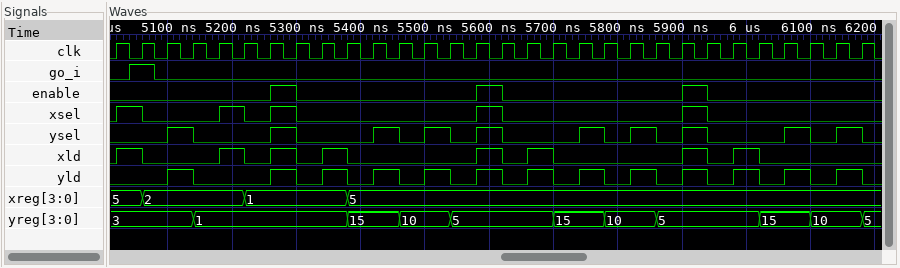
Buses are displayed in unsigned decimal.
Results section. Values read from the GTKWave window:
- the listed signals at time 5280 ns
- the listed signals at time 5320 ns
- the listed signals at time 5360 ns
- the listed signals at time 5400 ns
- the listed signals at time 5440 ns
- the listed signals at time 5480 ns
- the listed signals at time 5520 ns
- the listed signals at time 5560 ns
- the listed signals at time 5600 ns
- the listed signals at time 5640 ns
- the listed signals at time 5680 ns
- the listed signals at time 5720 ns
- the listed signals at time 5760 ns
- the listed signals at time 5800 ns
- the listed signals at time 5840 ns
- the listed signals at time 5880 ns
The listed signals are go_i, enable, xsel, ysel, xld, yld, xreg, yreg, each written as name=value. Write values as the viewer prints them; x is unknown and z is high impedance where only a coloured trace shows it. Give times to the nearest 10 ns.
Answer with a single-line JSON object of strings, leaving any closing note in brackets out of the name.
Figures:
{"the listed signals at time 5280 ns": "go_i=0, enable=1, xsel=1, ysel=1, xld=1, yld=1, xreg=1, yreg=1", "the listed signals at time 5320 ns": "go_i=0, enable=0, xsel=0, ysel=0, xld=0, yld=0, xreg=1, yreg=1", "the listed signals at time 5360 ns": "go_i=0, enable=0, xsel=0, ysel=0, xld=1, yld=1, xreg=1, yreg=1", "the listed signals at time 5400 ns": "go_i=0, enable=0, xsel=0, ysel=0, xld=0, yld=0, xreg=5, yreg=15", "the listed signals at time 5440 ns": "go_i=0, enable=0, xsel=0, ysel=1, xld=0, yld=1, xreg=5, yreg=15", "the listed signals at time 5480 ns": "go_i=0, enable=0, xsel=0, ysel=0, xld=0, yld=0, xreg=5, yreg=10", "the listed signals at time 5520 ns": "go_i=0, enable=0, xsel=0, ysel=1, xld=0, yld=1, xreg=5, yreg=10", "the listed signals at time 5560 ns": "go_i=0, enable=0, xsel=0, ysel=0, xld=0, yld=0, xreg=5, yreg=5", "the listed signals at time 5600 ns": "go_i=0, enable=1, xsel=1, ysel=1, xld=1, yld=1, xreg=5, yreg=5", "the listed signals at time 5640 ns": "go_i=0, enable=0, xsel=0, ysel=0, xld=0, yld=0, xreg=5, yreg=5", "the listed signals at time 5680 ns": "go_i=0, enable=0, xsel=0, ysel=0, xld=1, yld=1, xreg=5, yreg=5", "the listed signals at time 5720 ns": "go_i=0, enable=0, xsel=0, ysel=0, xld=0, yld=0, xreg=5, yreg=15", "the listed signals at time 5760 ns": "go_i=0, enable=0, xsel=0, ysel=1, xld=0, yld=1, xreg=5, yreg=15", "the listed signals at time 5800 ns": "go_i=0, enable=0, xsel=0, ysel=0, xld=0, yld=0, xreg=5, yreg=10", "the listed signals at time 5840 ns": "go_i=0, enable=0, xsel=0, ysel=1, xld=0, yld=1, xreg=5, yreg=10", "the listed signals at time 5880 ns": "go_i=0, enable=0, xsel=0, ysel=0, xld=0, yld=0, xreg=5, yreg=5"}
